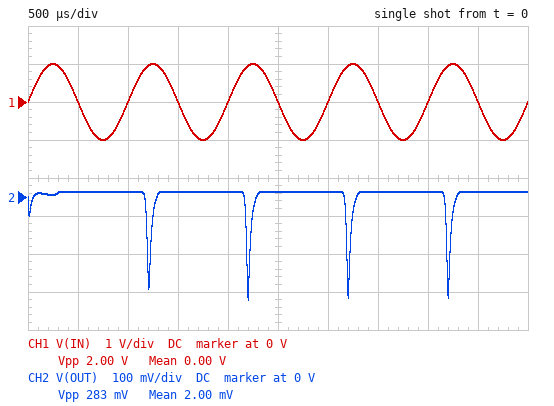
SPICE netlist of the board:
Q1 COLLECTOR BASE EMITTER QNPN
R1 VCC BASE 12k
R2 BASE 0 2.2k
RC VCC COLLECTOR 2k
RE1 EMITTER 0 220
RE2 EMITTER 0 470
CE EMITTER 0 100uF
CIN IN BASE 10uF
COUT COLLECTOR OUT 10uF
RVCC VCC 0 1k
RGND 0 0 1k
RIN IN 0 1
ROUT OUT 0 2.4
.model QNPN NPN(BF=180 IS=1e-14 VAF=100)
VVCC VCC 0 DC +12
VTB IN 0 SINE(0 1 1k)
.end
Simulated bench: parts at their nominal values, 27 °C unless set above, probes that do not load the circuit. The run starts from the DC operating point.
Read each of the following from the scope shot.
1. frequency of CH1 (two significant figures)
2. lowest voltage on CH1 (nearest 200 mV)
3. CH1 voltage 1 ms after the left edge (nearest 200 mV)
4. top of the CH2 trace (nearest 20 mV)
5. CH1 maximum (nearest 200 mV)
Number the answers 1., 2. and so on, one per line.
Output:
1. 1.0 kHz
2. -1.0 V
3. 0 V
4. 20 mV
5. 1.0 V
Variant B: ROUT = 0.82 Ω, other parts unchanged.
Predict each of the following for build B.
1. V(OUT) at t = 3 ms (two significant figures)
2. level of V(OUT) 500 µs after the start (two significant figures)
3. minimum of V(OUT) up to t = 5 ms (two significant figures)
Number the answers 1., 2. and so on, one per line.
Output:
1. 4.4 mV
2. 4.5 mV
3. -100 mV
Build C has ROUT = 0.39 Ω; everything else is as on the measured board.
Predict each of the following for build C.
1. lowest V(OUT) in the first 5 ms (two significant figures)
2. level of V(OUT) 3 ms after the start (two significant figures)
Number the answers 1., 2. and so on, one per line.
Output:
1. -49 mV
2. 2.1 mV
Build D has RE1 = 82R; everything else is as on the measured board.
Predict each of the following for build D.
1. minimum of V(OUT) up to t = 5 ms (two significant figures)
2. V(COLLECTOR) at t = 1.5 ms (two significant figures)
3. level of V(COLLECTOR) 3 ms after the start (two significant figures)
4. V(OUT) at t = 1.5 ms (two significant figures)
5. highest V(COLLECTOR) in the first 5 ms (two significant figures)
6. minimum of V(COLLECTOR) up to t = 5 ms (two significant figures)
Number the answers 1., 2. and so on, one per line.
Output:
1. -300 mV
2. 680 mV
3. 960 mV
4. 14 mV
5. 1.0 V
6. 460 mV
